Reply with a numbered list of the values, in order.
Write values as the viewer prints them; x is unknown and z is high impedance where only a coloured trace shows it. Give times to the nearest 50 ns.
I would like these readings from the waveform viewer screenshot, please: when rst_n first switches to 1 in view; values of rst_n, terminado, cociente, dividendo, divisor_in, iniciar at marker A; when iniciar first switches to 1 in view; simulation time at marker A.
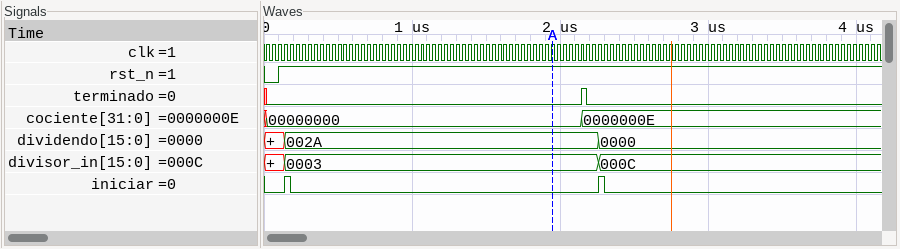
1. 100 ns
2. rst_n=1, terminado=0, cociente=00000000, dividendo=002A, divisor_in=0003, iniciar=0
3. 150 ns
4. 1950 ns
